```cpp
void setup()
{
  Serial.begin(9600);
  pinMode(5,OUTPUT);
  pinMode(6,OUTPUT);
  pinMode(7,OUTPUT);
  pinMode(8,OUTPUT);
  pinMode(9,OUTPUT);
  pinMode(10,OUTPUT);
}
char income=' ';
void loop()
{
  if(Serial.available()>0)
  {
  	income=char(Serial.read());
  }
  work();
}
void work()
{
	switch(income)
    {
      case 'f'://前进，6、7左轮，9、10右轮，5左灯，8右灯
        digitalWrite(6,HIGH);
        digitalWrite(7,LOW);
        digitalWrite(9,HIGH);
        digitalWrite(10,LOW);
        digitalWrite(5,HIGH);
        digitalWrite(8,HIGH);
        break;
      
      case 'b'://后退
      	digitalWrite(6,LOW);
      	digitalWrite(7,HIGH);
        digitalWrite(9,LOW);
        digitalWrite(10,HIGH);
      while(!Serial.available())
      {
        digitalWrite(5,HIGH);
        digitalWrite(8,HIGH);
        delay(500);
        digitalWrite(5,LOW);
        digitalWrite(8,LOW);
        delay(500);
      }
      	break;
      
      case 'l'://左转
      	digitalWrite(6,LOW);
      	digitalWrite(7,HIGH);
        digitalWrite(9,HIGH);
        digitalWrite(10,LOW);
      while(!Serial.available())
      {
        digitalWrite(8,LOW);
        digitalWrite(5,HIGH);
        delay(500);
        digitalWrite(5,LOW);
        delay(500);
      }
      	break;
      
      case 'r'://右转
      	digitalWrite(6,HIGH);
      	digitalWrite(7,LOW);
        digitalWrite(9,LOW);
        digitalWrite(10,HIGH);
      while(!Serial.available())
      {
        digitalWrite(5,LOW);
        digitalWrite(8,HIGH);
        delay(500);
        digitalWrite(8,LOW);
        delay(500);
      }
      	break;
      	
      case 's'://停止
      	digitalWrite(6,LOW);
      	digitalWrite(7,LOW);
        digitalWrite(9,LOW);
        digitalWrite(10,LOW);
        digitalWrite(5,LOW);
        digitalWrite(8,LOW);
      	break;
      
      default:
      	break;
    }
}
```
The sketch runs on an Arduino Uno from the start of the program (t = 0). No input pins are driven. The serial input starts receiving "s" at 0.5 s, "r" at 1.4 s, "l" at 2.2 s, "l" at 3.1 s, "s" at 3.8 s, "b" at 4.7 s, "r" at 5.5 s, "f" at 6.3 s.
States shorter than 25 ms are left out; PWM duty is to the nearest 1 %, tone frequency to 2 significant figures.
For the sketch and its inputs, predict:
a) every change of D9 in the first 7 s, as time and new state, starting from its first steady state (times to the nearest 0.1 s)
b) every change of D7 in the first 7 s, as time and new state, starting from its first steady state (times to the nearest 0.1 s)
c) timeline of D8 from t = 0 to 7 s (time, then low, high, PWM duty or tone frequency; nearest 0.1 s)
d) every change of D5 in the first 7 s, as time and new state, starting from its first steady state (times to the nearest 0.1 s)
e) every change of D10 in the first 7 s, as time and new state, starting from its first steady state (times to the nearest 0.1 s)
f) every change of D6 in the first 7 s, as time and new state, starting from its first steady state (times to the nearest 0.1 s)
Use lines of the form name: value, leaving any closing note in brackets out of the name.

every change of D9 in the first 7 s, as time and new state, starting from its first steady state: 0 s low; 2.4 s high; 4.4 s low; 6.7 s high
every change of D7 in the first 7 s, as time and new state, starting from its first steady state: 0 s low; 2.4 s high; 4.4 s low; 4.7 s high; 5.7 s low
timeline of D8 from t = 0 to 7 s: 0 s low; 1.4 s high; 1.9 s low; 4.7 s high; 5.2 s low; 5.7 s high; 6.2 s low; 6.7 s high
every change of D5 in the first 7 s, as time and new state, starting from its first steady state: 0 s low; 2.4 s high; 2.9 s low; 3.4 s high; 3.9 s low; 4.7 s high; 5.2 s low; 6.7 s high
every change of D10 in the first 7 s, as time and new state, starting from its first steady state: 0 s low; 1.4 s high; 2.4 s low; 4.7 s high; 6.7 s low
every change of D6 in the first 7 s, as time and new state, starting from its first steady state: 0 s low; 1.4 s high; 2.4 s low; 5.7 s high
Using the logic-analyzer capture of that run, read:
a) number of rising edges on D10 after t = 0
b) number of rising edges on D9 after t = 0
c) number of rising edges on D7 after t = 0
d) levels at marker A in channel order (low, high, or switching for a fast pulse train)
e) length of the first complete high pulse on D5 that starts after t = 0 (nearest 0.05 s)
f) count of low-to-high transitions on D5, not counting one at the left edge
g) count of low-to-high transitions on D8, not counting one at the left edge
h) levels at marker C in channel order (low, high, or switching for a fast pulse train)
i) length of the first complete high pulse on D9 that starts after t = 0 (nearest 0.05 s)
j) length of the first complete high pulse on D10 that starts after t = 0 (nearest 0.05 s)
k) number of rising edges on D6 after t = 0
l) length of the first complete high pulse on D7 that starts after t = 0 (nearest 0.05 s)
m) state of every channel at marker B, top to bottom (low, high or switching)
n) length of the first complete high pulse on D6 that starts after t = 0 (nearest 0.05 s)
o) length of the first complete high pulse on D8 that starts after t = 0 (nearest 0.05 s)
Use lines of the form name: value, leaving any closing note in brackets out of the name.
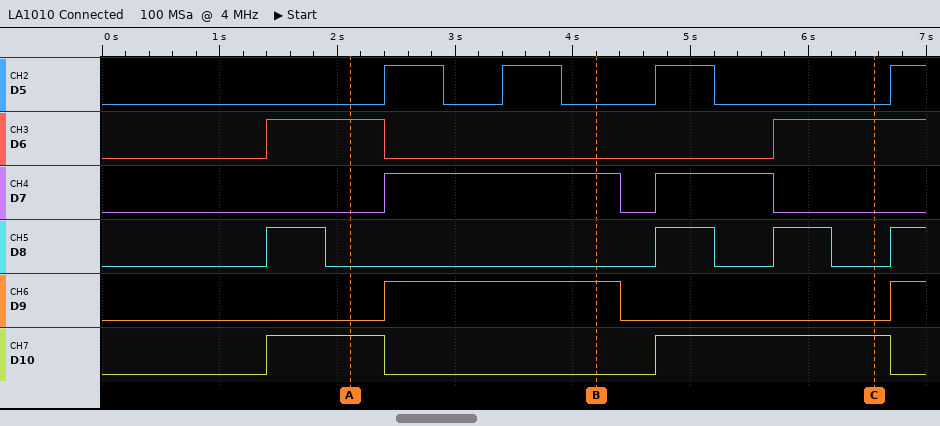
number of rising edges on D10 after t = 0: 2
number of rising edges on D9 after t = 0: 2
number of rising edges on D7 after t = 0: 2
levels at marker A in channel order: D5 low, D6 high, D7 low, D8 low, D9 low, D10 high
length of the first complete high pulse on D5 that starts after t = 0: 0.50 s
count of low-to-high transitions on D5, not counting one at the left edge: 4
count of low-to-high transitions on D8, not counting one at the left edge: 4
levels at marker C in channel order: D5 low, D6 high, D7 low, D8 low, D9 low, D10 high
length of the first complete high pulse on D9 that starts after t = 0: 2.00 s
length of the first complete high pulse on D10 that starts after t = 0: 1.00 s
number of rising edges on D6 after t = 0: 2
length of the first complete high pulse on D7 that starts after t = 0: 2.00 s
state of every channel at marker B, top to bottom: D5 low, D6 low, D7 high, D8 low, D9 high, D10 low
length of the first complete high pulse on D6 that starts after t = 0: 1.00 s
length of the first complete high pulse on D8 that starts after t = 0: 0.50 s
